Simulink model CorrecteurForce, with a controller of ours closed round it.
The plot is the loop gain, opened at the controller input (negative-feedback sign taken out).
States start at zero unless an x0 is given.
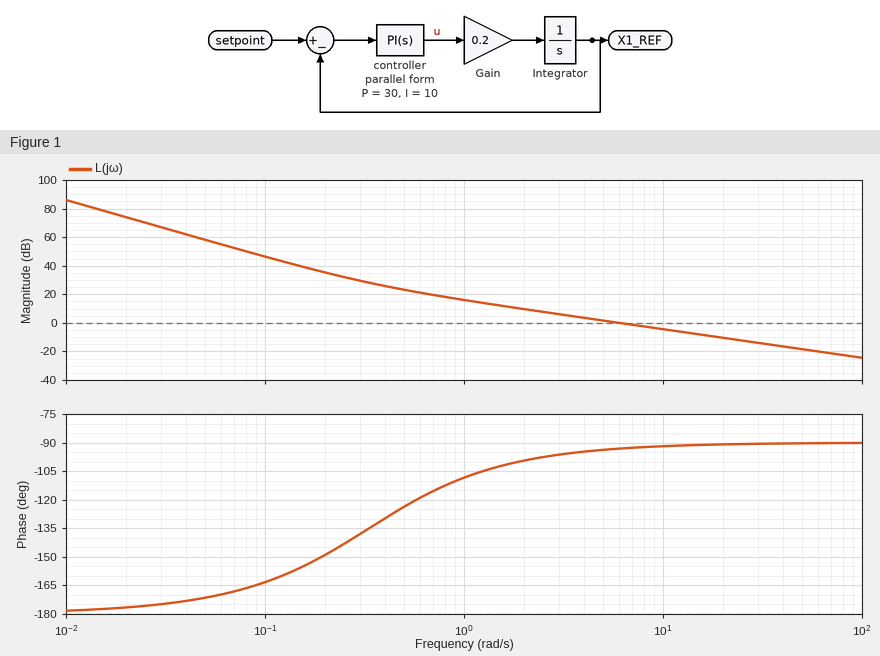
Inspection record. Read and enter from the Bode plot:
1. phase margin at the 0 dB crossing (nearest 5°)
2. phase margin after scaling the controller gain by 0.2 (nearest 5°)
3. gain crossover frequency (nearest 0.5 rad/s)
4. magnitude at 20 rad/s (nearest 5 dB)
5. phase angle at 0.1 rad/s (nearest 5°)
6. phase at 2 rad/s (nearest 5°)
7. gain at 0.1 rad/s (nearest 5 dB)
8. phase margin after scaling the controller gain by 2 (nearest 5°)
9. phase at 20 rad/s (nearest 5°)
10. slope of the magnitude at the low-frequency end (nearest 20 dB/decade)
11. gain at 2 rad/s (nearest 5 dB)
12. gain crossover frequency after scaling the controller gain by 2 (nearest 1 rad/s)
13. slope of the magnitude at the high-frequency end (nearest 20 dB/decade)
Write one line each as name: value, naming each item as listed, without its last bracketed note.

phase margin at the 0 dB crossing: 85°
phase margin after scaling the controller gain by 0.2: 75°
gain crossover frequency: 6.0 rad/s
magnitude at 20 rad/s: -10 dB
phase angle at 0.1 rad/s: -165°
phase at 2 rad/s: -100°
gain at 0.1 rad/s: 45 dB
phase margin after scaling the controller gain by 2: 90°
phase at 20 rad/s: -90°
slope of the magnitude at the low-frequency end: -40 dB/decade
gain at 2 rad/s: 10 dB
gain crossover frequency after scaling the controller gain by 2: 12 rad/s
slope of the magnitude at the high-frequency end: -20 dB/decade
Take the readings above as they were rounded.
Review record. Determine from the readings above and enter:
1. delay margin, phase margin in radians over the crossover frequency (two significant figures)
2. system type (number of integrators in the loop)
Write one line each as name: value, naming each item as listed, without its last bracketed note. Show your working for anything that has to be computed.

delay margin, phase margin in radians over the crossover frequency: 85 × π / 180 / 6 = 0.25 s
system type: 2
